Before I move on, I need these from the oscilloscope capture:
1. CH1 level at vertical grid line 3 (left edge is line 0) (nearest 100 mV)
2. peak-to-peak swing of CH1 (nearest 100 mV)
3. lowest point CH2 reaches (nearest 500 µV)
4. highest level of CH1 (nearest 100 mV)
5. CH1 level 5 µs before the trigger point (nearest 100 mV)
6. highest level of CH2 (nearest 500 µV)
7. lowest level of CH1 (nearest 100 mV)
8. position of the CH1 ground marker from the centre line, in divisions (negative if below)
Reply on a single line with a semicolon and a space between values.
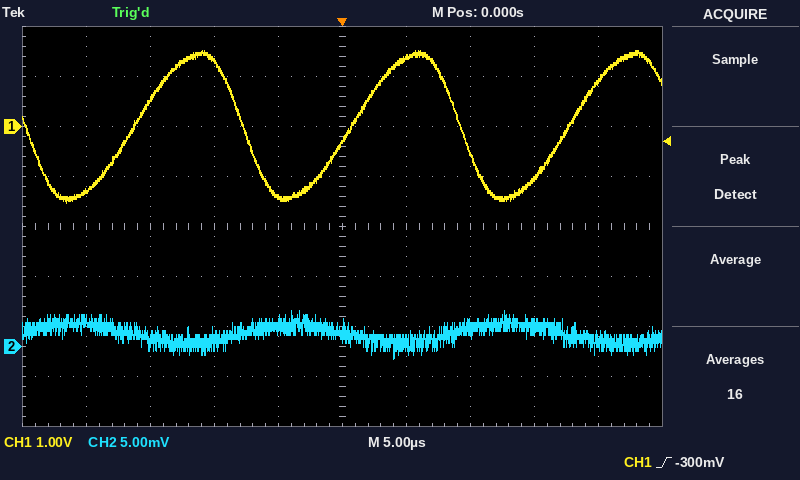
1.3 V; 3.0 V; -1.0 mV; 1.5 V; -1.4 V; 3.5 mV; -1.5 V; +2.0 div
